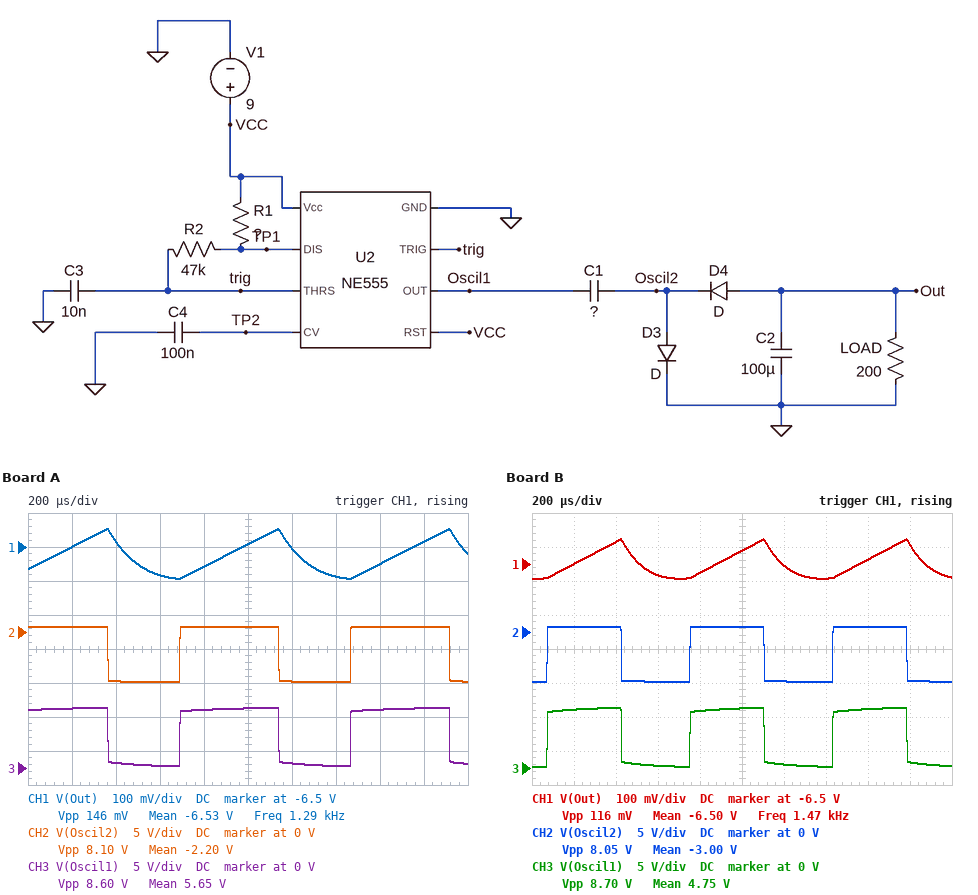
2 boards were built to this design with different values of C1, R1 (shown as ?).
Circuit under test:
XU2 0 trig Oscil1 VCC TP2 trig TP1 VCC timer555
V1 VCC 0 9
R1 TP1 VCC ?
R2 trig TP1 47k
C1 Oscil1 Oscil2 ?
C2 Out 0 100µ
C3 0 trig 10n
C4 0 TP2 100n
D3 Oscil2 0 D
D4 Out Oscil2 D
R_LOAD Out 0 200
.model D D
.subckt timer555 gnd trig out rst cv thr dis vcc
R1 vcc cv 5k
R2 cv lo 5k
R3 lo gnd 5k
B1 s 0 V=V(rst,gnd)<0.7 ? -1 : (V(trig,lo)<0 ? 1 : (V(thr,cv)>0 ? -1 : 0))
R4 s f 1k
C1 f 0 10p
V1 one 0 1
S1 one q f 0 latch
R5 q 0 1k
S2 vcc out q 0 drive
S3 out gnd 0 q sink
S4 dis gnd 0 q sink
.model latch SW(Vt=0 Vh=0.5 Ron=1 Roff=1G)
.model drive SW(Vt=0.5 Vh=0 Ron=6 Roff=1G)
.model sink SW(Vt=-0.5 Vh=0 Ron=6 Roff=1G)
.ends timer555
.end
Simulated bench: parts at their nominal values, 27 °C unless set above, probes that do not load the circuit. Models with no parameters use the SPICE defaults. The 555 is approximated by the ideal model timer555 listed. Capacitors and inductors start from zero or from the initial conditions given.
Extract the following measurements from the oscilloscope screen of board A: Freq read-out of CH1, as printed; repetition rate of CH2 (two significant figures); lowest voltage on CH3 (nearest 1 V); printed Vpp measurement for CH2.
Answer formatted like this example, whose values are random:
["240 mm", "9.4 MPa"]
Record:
["1.29 kHz", "1.3 kHz", "0 V", "8.10 V"]
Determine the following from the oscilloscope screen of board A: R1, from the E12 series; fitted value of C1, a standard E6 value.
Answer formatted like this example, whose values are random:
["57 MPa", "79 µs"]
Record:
["18 kΩ", "47 µF"]
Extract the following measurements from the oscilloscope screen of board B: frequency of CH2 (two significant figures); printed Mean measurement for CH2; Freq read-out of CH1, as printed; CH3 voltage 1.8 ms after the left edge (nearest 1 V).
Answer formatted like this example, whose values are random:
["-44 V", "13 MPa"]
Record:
["1.5 kHz", "-3.00 V", "1.47 kHz", "1 V"]
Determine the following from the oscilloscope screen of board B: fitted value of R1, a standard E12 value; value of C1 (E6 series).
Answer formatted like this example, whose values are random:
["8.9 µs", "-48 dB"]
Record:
["3.9 kΩ", "33 µF"]
